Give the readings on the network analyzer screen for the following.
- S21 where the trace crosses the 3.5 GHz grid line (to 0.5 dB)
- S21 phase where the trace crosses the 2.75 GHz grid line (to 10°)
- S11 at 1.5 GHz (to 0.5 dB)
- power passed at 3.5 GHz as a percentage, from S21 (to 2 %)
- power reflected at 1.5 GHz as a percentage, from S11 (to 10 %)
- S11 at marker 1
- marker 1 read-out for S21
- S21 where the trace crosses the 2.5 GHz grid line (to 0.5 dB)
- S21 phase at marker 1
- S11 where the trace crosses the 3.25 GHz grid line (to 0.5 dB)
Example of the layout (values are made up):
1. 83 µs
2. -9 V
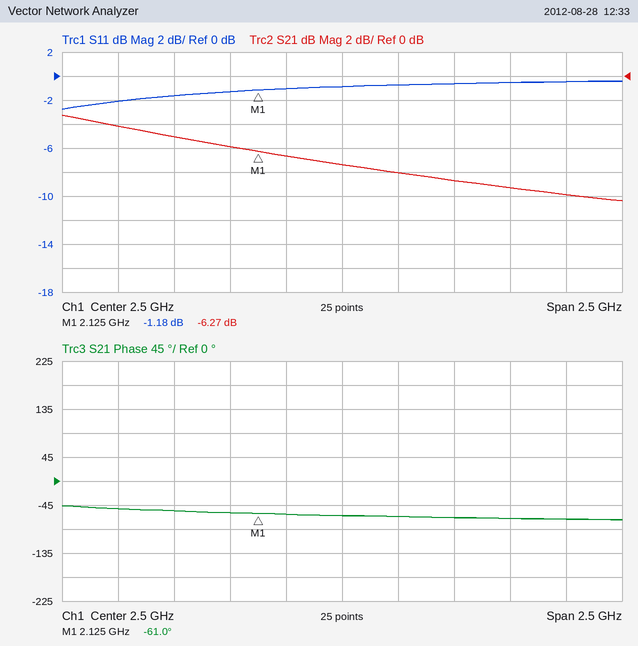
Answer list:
1. -10.0 dB
2. -70°
3. -2.0 dB
4. 10 %
5. 60 %
6. -1.18 dB
7. -6.27 dB
8. -7.5 dB
9. -61.0°
10. -0.5 dB
